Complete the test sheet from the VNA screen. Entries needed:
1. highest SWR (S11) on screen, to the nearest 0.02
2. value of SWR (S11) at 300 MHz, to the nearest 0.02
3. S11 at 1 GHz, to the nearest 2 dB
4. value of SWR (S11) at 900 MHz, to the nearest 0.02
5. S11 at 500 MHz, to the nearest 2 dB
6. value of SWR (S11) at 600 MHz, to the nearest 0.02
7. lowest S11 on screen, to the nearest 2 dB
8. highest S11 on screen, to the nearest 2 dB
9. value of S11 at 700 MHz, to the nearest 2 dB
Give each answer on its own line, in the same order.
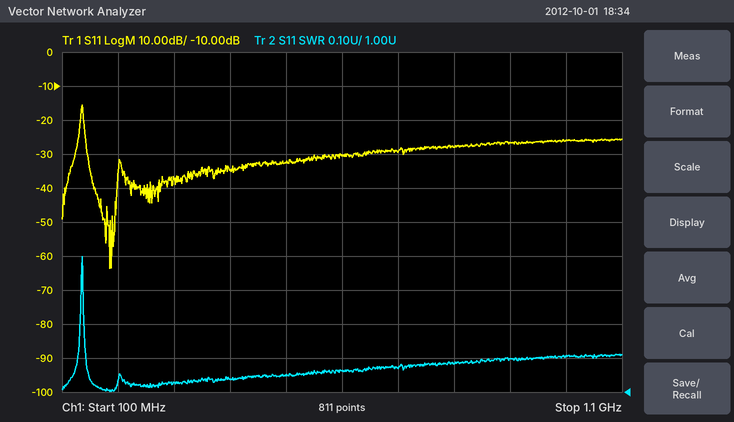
1.40
1.02
-26 dB
1.10
-32 dB
1.06
-64 dB
-16 dB
-30 dB
